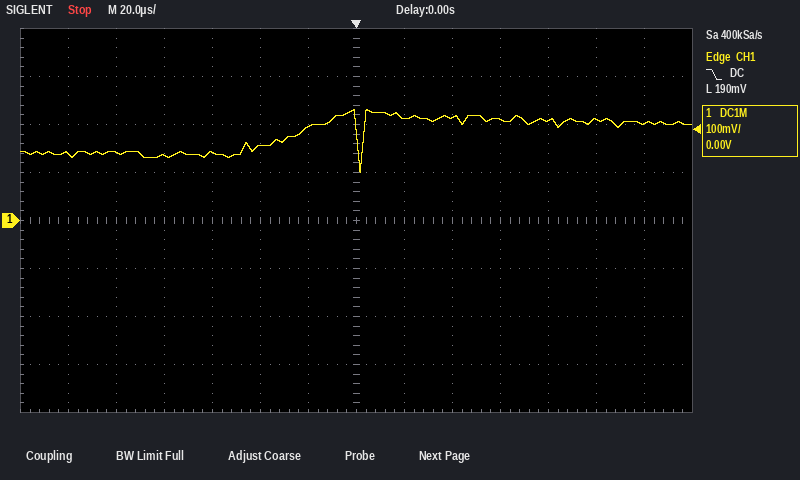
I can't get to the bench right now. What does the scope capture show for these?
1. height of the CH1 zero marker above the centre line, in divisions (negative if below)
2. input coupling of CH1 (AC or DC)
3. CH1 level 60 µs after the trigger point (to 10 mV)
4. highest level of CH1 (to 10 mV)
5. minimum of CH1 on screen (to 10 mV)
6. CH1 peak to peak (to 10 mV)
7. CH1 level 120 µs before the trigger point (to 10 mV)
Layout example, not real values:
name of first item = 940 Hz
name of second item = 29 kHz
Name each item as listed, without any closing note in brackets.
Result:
height of the CH1 zero marker above the centre line, in divisions = 0.0 div
input coupling of CH1 = DC
CH1 level 60 µs after the trigger point = 210 mV
highest level of CH1 = 230 mV
minimum of CH1 on screen = 100 mV
CH1 peak to peak = 130 mV
CH1 level 120 µs before the trigger point = 140 mV
